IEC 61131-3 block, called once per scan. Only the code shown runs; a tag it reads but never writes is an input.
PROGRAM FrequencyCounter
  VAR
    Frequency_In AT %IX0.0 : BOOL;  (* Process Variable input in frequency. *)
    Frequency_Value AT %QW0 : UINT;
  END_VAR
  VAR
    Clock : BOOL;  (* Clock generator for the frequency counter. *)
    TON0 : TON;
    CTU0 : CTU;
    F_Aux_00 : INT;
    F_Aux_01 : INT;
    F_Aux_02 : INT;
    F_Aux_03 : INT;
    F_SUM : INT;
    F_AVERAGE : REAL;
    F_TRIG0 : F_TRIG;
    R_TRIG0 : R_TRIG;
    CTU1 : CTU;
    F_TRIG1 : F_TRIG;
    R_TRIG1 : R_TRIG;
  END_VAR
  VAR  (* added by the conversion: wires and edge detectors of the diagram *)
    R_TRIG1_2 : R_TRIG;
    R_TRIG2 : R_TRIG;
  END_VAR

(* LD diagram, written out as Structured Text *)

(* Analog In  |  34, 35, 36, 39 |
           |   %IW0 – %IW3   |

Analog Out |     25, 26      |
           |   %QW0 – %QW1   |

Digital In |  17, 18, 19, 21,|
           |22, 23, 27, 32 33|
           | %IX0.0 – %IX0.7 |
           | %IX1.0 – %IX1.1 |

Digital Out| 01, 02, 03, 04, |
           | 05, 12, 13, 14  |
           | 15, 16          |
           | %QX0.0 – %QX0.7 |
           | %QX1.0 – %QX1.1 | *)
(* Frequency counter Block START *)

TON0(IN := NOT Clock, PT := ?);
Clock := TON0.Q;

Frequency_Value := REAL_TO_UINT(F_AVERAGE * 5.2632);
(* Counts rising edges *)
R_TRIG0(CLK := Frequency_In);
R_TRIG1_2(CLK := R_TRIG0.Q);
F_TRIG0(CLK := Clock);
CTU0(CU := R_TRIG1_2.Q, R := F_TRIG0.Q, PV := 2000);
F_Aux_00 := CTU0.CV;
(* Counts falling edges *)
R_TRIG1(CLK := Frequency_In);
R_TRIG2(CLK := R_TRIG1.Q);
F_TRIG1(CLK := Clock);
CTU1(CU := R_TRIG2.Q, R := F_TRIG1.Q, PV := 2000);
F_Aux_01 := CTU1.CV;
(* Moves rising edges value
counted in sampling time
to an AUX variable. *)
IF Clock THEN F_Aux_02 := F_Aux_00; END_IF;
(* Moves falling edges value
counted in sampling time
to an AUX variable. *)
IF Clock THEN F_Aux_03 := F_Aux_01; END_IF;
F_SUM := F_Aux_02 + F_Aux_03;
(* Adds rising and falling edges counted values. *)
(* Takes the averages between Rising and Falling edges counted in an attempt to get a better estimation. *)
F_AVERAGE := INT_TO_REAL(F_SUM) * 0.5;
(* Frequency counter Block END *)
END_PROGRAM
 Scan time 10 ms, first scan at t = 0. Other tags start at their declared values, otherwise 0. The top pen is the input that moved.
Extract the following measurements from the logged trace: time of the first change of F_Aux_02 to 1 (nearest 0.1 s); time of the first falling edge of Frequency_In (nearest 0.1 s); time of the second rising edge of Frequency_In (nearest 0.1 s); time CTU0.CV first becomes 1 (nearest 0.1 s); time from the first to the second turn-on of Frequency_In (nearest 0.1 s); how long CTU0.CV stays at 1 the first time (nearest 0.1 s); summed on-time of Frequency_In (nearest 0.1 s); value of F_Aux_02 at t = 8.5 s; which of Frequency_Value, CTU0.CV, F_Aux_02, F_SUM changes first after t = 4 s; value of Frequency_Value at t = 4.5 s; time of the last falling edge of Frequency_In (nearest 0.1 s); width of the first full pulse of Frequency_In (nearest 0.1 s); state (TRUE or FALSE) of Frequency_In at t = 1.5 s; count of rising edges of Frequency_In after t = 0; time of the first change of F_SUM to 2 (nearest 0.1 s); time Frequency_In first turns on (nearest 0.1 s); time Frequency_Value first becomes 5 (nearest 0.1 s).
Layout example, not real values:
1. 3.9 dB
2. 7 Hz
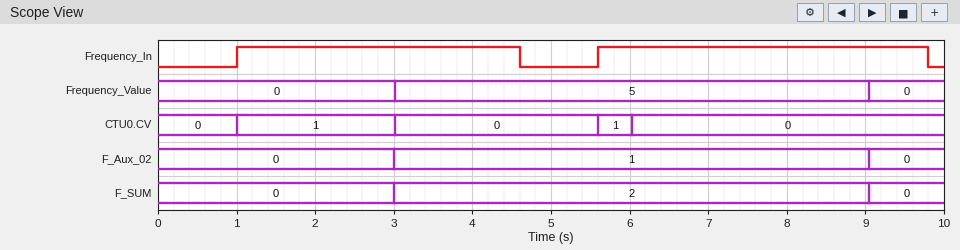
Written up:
1. 3.0 s
2. 4.6 s
3. 5.6 s
4. 1.0 s
5. 4.6 s
6. 2.0 s
7. 7.8 s
8. 1
9. CTU0.CV
10. 5
11. 9.8 s
12. 3.6 s
13. TRUE
14. 2
15. 3.0 s
16. 1.0 s
17. 3.0 s
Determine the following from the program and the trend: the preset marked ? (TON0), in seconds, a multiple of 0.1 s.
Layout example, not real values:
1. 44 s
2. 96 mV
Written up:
1. 3.0 s
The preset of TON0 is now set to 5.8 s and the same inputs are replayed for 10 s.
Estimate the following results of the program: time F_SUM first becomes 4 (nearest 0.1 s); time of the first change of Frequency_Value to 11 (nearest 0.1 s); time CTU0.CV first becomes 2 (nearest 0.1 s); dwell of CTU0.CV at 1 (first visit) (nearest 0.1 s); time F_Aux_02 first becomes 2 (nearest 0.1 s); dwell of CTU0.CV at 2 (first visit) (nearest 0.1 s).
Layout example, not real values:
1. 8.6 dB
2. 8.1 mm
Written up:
1. 5.8 s
2. 5.8 s
3. 5.6 s
4. 4.6 s
5. 5.8 s
6. 0.2 s
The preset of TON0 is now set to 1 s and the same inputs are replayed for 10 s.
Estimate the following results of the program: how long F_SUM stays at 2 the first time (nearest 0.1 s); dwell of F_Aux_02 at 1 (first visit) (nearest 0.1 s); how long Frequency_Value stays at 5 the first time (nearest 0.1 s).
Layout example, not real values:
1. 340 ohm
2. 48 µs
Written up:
1. 1.0 s
2. 1.0 s
3. 1.0 s
